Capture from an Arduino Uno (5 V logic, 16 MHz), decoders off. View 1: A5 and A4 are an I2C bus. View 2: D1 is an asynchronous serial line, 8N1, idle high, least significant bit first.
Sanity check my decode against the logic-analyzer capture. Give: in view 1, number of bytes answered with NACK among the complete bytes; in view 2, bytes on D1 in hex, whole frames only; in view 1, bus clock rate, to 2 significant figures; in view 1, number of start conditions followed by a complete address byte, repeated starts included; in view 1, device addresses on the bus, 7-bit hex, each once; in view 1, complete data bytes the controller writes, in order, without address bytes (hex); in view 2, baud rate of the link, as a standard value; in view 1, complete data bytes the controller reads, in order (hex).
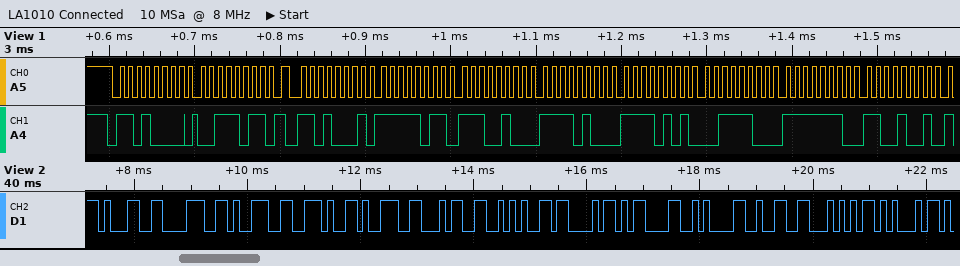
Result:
0
0x31 0x38 0x39 0x2E 0x39 0x34 0x2A 0x43 0x0D 0x0A 0x32 0x54 0x45
100 kHz
2
0x68
3B
9600 baud
FB E4 F4 F5 3C FE C9
